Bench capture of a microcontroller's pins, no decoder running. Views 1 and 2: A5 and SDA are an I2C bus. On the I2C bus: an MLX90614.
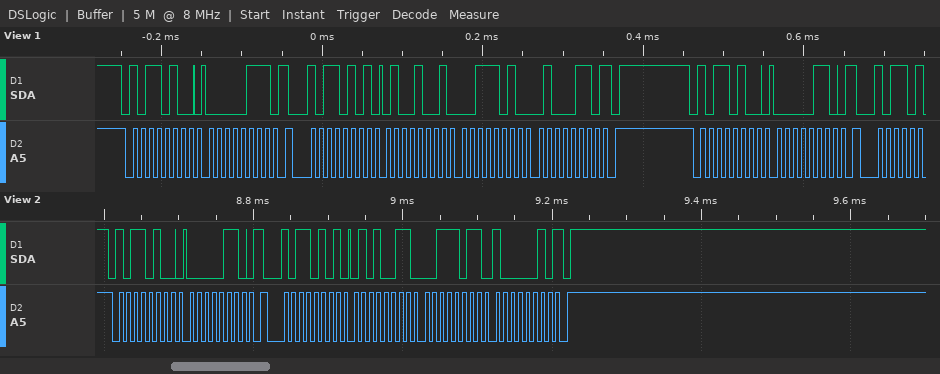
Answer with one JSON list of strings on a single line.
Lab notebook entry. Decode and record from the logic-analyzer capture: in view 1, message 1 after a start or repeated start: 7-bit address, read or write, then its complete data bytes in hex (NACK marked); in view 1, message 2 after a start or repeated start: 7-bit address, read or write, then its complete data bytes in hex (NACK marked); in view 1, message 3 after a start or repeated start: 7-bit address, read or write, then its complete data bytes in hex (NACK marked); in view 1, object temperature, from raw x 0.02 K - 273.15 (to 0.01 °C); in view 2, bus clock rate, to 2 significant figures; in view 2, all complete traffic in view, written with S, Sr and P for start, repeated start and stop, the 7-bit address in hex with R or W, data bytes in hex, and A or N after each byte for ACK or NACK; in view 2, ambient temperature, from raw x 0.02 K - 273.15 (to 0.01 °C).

["0x5A write: 07", "0x5A read: 49 3A 46 NACK", "0x5A write: 06", "25.27 °C", "100 kHz", "S 5AW A 06 A Sr 5AR A 53 A 3B A 82 N P", "30.59 °C"]
